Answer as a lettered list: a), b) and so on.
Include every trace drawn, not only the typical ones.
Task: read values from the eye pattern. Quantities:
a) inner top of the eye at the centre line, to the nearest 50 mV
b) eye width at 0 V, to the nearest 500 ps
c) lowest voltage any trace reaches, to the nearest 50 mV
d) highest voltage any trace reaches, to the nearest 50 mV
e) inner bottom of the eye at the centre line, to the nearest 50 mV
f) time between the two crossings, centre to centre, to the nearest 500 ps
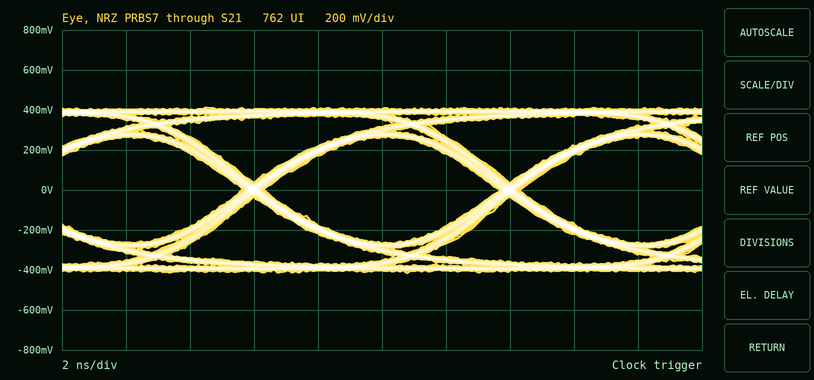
a) 250 mV
b) 7.5 ns
c) -400 mV
d) 400 mV
e) -250 mV
f) 8.0 ns
